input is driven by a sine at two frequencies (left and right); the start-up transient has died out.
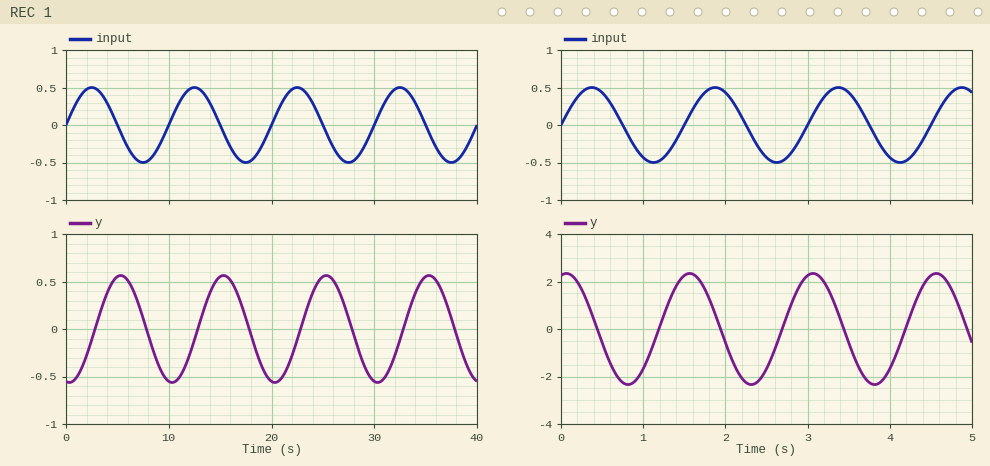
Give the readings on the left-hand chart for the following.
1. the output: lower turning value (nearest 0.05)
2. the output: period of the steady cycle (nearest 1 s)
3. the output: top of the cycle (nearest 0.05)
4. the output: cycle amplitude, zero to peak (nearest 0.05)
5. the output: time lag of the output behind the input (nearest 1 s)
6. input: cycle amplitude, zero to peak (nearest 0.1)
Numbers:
-0.55
10 s
0.55
0.55
3 s
0.5
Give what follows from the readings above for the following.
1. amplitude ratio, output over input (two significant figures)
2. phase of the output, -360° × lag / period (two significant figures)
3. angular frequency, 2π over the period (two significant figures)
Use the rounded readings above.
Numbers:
1.1
-110°
0.63 rad/s
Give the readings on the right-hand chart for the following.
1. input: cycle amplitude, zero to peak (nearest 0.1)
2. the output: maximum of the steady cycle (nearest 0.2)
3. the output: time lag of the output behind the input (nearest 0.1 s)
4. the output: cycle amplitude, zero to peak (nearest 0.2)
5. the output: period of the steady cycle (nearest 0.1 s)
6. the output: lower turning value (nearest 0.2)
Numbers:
0.5
2.4
1.2 s
2.4
1.5 s
-2.4
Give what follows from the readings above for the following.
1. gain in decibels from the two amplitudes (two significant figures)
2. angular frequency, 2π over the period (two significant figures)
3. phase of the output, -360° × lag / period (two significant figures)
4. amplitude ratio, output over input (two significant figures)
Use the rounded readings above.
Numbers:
14 dB
4.2 rad/s
-290°
4.8
